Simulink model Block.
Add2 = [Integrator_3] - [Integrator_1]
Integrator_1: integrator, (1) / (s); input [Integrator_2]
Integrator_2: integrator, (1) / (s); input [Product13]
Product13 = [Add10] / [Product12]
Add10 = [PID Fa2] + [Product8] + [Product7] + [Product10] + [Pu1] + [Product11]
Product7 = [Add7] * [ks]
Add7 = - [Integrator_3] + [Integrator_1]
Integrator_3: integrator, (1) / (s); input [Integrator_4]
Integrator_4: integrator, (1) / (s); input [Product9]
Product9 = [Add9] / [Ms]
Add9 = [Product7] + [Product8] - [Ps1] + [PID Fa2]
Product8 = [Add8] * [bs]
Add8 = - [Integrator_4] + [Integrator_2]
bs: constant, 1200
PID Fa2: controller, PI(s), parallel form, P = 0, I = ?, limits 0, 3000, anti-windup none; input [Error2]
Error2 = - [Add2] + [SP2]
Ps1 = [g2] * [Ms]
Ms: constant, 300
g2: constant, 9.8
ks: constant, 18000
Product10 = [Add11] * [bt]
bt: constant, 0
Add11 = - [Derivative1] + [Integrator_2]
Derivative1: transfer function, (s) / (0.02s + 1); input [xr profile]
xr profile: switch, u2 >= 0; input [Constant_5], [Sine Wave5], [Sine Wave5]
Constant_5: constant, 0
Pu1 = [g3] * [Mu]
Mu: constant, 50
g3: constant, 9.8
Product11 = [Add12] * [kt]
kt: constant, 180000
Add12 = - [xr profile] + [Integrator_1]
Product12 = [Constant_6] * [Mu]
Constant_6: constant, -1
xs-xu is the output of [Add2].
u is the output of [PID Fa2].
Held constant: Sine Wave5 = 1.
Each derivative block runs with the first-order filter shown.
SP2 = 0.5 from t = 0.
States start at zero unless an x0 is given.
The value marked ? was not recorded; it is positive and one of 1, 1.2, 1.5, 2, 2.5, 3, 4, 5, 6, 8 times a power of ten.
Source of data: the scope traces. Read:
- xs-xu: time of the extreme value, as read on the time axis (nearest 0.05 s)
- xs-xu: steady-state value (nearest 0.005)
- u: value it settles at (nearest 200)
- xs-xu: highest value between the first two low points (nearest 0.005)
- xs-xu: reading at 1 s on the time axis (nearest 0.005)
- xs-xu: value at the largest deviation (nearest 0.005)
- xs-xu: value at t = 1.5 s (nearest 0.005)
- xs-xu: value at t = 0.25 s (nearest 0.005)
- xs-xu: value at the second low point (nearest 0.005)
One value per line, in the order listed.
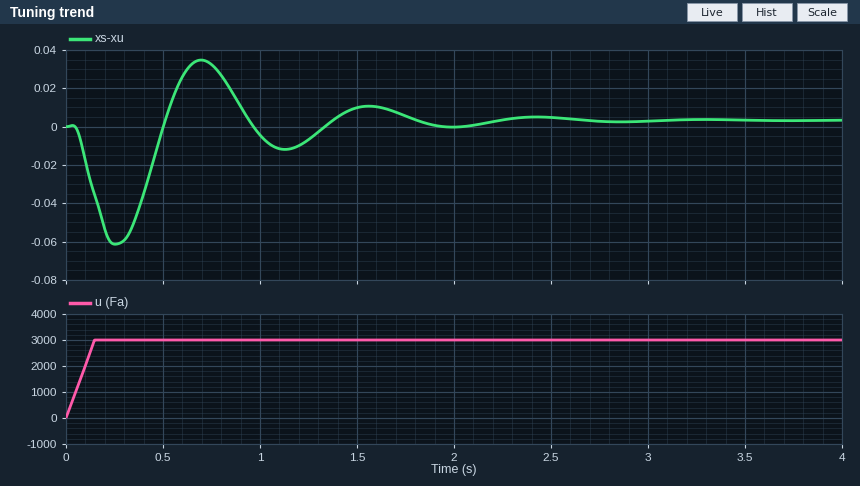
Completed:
0.25 s
0.005
3000
0.035
-0.005
-0.060
0.010
-0.060
-0.010
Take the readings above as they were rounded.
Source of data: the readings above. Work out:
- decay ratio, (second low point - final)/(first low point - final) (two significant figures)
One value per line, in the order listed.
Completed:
0.23
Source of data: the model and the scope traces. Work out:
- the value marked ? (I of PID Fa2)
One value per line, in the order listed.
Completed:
40000
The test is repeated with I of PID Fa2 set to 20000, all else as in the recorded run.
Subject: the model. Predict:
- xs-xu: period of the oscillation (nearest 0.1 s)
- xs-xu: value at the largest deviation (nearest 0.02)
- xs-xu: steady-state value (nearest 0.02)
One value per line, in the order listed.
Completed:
0.9 s
-0.10
0.00
